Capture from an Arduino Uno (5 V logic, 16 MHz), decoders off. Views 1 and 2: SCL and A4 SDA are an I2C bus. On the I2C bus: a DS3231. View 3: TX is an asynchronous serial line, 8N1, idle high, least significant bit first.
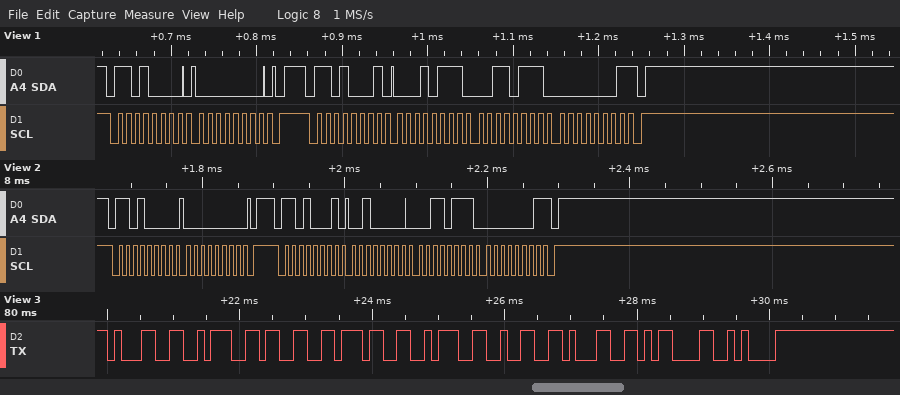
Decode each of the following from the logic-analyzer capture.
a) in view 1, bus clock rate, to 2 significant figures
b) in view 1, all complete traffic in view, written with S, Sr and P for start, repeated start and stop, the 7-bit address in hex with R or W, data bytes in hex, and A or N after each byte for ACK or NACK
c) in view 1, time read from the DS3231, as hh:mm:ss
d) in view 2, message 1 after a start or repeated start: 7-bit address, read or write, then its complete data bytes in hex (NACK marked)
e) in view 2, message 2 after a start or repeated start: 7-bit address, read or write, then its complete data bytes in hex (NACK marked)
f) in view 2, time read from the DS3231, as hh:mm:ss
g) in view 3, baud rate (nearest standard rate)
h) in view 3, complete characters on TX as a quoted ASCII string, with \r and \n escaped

100 kHz
S 68W A 00 A P S 68R A 17 A 37 A 01 N P
01:37:17
0x68 write: 00
0x68 read: 20 37 01 NACK
01:37:20
9600 baud
"1:37:21\r\n"
